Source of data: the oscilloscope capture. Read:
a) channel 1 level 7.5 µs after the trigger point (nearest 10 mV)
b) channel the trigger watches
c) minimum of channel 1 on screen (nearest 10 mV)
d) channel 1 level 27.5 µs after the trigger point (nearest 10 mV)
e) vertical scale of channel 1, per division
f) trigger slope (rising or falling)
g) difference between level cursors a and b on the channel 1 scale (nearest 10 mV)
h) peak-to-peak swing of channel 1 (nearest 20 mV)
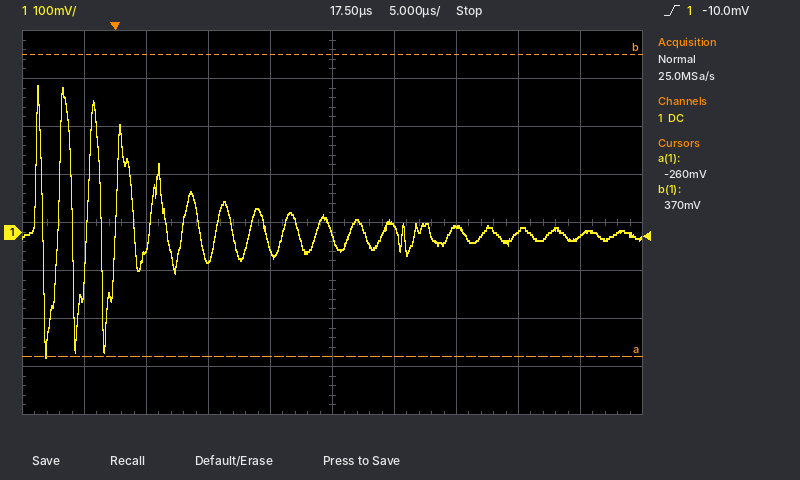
-60 mV
channel 1
-260 mV
10 mV
100 mV
rising
630 mV
560 mV
